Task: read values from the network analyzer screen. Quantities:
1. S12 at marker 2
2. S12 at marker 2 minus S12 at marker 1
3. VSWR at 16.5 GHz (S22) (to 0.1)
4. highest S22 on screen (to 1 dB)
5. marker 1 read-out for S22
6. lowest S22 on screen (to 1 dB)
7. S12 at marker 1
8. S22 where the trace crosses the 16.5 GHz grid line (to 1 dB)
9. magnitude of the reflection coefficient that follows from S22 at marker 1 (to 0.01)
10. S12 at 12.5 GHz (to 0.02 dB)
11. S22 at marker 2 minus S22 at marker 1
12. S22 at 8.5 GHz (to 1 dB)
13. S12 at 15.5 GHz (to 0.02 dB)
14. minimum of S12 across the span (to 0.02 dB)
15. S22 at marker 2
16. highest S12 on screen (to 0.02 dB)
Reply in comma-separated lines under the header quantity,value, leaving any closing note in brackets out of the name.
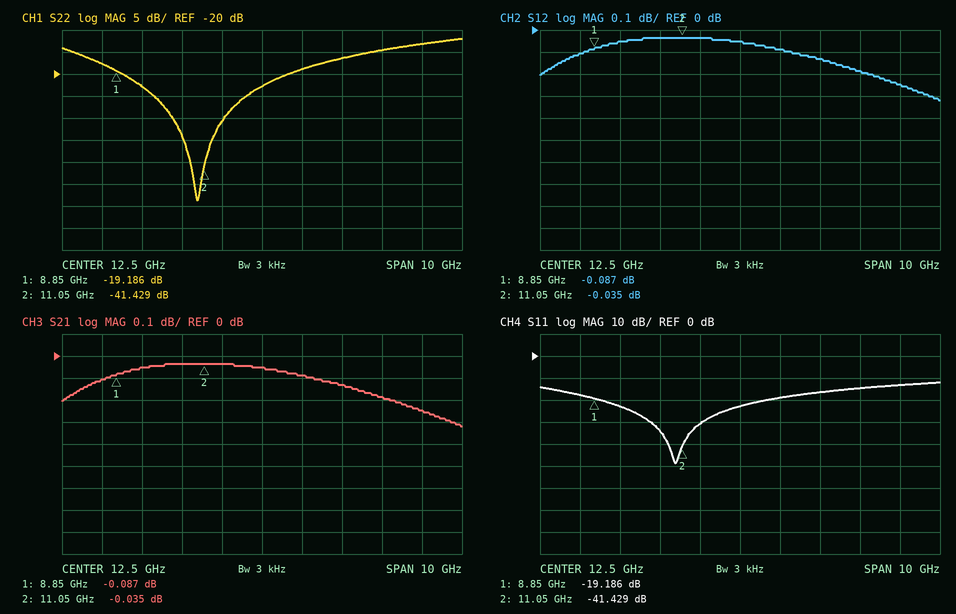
quantity,value
S12 at marker 2,-0.035 dB
S12 at marker 2 minus S12 at marker 1,0.052 dB
VSWR at 16.5 GHz (S22),1.6
highest S22 on screen,-12 dB
marker 1 read-out for S22,-19.186 dB
lowest S22 on screen,-49 dB
S12 at marker 1,-0.087 dB
S22 where the trace crosses the 16.5 GHz grid line,-13 dB
magnitude of the reflection coefficient that follows from S22 at marker 1,0.11
S12 at 12.5 GHz,-0.06 dB
S22 at marker 2 minus S22 at marker 1,-22.243 dB
S22 at 8.5 GHz,-18 dB
S12 at 15.5 GHz,-0.18 dB
minimum of S12 across the span,-0.32 dB
S22 at marker 2,-41.429 dB
highest S12 on screen,-0.04 dB
